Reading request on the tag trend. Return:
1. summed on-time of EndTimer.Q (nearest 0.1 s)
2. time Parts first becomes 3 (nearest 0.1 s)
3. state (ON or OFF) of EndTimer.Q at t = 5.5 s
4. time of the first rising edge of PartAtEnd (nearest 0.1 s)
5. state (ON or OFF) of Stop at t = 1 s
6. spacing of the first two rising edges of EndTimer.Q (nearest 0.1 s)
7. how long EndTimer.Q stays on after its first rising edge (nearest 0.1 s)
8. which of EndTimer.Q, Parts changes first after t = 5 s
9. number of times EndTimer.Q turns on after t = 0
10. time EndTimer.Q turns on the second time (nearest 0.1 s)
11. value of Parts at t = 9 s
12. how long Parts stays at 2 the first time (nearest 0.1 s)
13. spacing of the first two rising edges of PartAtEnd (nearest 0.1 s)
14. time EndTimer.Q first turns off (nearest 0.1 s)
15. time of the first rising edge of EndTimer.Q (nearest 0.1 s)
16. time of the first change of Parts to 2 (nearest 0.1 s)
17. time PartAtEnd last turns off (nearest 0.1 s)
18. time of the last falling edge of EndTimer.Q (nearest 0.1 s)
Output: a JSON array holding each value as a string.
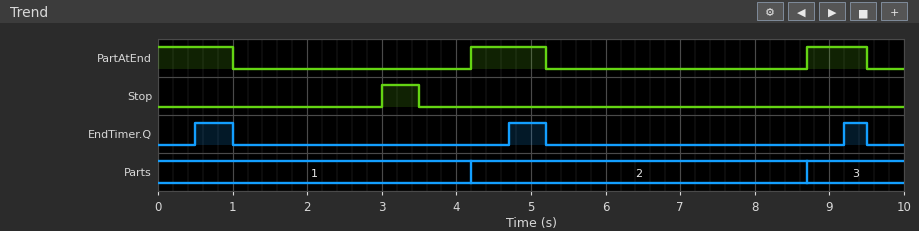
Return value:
["1.3 s", "8.7 s", "OFF", "4.2 s", "OFF", "4.2 s", "0.5 s", "EndTimer.Q", "3", "4.7 s", "3", "4.5 s", "4.5 s", "1.0 s", "0.5 s", "4.2 s", "9.5 s", "9.5 s"]
